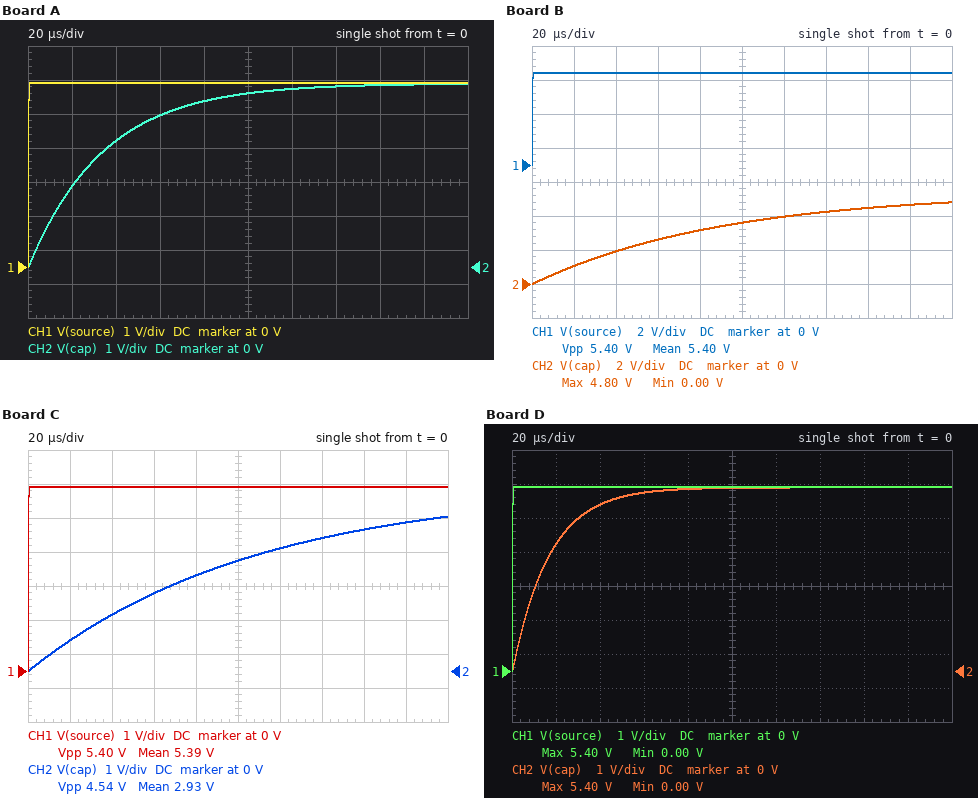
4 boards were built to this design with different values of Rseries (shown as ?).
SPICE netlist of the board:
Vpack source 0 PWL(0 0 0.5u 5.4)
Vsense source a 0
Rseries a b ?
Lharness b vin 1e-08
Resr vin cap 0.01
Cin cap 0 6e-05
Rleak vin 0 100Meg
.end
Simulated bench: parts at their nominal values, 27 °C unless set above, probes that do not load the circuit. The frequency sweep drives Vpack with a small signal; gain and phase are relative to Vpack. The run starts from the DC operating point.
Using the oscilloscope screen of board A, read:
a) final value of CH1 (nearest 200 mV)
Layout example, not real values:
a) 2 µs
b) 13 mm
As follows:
a) 5.4 V
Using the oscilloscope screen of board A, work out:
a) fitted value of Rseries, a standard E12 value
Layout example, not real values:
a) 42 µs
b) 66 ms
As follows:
a) 0.56 Ω
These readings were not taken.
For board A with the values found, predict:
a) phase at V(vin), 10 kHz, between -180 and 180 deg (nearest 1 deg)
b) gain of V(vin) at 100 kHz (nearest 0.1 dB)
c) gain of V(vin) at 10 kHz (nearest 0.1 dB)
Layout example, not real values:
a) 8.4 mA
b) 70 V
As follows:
a) -63 deg
b) -26.1 dB
c) -7.5 dB
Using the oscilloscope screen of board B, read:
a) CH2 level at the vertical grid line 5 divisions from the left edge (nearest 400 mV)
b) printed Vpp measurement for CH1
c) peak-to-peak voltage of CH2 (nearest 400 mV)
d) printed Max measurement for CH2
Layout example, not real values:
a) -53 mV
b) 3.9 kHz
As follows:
a) 3.6 V
b) 5.40 V
c) 4.8 V
d) 4.80 V
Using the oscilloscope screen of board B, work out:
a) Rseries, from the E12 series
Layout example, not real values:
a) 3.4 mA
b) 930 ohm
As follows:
a) 1.5 Ω
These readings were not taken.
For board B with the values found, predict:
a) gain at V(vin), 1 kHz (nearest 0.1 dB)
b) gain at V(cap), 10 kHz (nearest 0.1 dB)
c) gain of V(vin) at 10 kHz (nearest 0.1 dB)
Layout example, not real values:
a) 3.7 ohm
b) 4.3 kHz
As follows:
a) -1.2 dB
b) -15.2 dB
c) -15.2 dB
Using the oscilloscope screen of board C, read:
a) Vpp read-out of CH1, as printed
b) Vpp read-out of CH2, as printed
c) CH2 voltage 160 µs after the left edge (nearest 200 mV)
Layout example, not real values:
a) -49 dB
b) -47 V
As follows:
a) 5.40 V
b) 4.54 V
c) 4.2 V
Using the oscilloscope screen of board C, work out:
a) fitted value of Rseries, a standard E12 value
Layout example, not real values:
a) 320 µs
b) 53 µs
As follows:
a) 1.8 Ω
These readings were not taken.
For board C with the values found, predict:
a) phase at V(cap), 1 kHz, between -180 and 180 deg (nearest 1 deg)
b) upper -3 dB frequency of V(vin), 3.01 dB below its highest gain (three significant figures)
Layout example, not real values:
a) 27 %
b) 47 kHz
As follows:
a) -34 deg
b) 1.47 kHz
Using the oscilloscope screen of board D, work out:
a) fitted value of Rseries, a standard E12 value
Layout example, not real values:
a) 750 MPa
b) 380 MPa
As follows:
a) 0.27 Ω
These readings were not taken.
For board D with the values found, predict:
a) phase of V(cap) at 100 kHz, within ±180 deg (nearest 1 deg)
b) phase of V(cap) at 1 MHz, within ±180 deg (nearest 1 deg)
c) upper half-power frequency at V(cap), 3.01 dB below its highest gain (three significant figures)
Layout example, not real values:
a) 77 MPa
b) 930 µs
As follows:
a) -86 deg
b) -102 deg
c) 9.49 kHz
